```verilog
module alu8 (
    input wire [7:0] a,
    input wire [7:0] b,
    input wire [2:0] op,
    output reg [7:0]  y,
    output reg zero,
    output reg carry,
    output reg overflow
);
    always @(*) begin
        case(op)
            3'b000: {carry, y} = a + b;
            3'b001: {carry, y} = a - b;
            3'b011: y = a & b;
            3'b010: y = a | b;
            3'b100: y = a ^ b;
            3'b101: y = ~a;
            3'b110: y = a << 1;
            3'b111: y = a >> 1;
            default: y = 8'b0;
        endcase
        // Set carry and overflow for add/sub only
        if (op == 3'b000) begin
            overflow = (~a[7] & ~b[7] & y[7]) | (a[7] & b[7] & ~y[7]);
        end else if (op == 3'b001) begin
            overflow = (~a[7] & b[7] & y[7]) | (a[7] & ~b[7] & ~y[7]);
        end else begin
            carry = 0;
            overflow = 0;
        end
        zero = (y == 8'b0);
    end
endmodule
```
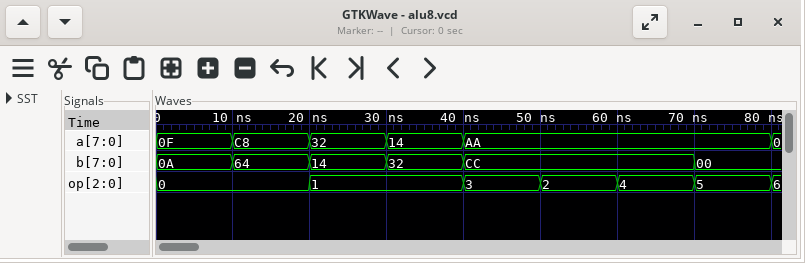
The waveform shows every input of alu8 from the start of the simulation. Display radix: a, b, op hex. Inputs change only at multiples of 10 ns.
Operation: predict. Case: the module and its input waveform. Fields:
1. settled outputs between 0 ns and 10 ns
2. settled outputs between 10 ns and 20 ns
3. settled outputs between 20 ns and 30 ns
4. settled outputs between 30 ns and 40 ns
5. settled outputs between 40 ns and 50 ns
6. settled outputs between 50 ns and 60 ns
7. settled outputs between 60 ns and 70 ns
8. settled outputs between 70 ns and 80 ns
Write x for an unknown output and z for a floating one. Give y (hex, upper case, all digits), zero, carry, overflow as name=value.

y=19, zero=0, carry=0, overflow=0
y=2C, zero=0, carry=1, overflow=0
y=1E, zero=0, carry=0, overflow=0
y=E2, zero=0, carry=1, overflow=0
y=88, zero=0, carry=0, overflow=0
y=EE, zero=0, carry=0, overflow=0
y=66, zero=0, carry=0, overflow=0
y=55, zero=0, carry=0, overflow=0
